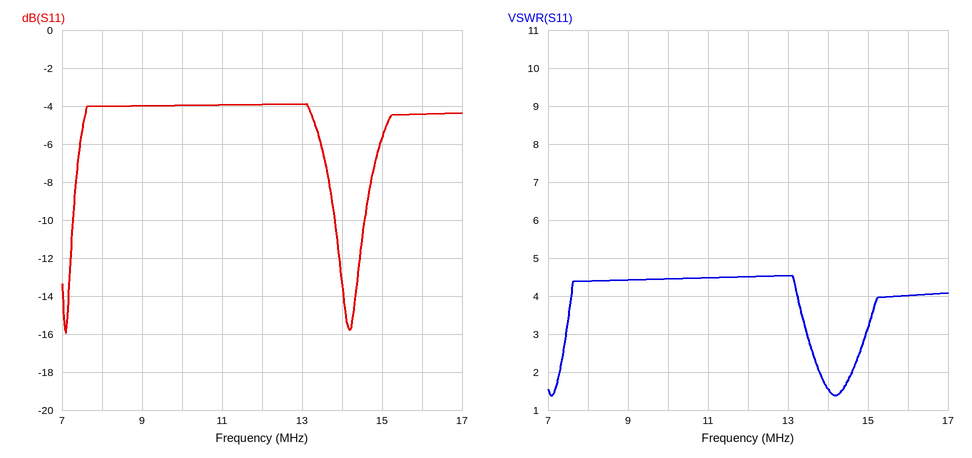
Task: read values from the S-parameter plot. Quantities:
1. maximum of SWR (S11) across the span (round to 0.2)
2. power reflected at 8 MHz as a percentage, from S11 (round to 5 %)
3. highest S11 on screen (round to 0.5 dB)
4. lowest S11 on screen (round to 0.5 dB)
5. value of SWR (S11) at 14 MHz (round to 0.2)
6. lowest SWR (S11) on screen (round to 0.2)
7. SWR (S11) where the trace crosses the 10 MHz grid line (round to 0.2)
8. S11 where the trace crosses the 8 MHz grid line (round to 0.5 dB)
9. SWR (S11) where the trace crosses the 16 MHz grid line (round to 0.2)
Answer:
4.6
40 %
-4.0 dB
-16.0 dB
1.6
1.4
4.4
-4.0 dB
4.0
